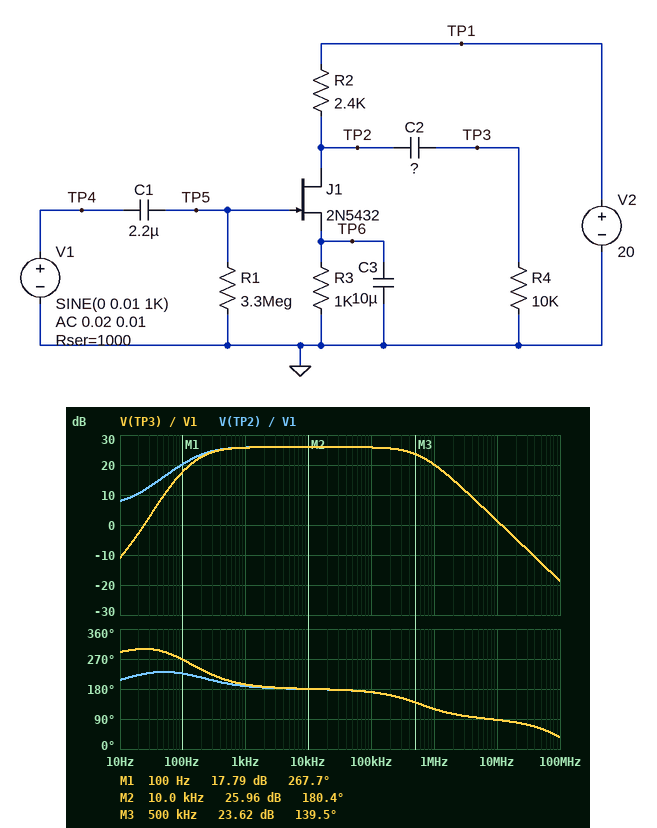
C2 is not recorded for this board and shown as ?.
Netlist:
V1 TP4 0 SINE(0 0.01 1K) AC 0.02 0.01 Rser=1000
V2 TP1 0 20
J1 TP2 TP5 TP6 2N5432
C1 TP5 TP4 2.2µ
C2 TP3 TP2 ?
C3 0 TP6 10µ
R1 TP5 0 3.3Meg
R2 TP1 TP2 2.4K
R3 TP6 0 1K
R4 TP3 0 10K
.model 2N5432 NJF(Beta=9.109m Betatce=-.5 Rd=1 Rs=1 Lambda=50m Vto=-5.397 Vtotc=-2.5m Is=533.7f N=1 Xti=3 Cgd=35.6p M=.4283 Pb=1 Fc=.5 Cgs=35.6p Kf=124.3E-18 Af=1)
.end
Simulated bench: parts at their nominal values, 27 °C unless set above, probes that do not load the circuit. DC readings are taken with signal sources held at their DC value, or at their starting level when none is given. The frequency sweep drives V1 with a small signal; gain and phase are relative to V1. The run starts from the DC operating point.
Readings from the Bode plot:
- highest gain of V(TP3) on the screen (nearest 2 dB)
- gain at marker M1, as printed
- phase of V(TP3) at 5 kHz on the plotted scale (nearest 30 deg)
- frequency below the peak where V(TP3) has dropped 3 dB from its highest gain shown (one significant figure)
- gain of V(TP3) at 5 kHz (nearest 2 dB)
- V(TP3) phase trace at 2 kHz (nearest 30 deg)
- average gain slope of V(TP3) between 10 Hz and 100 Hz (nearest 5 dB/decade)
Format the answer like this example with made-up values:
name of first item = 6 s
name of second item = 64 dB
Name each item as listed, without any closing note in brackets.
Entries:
highest gain of V(TP3) on the screen = 26 dB
gain at marker M1, as printed = 17.79 dB
phase of V(TP3) at 5 kHz on the plotted scale = 180 deg
frequency below the peak where V(TP3) has dropped 3 dB from its highest gain shown = 200 Hz
gain of V(TP3) at 5 kHz = 26 dB
V(TP3) phase trace at 2 kHz = 180 deg
average gain slope of V(TP3) between 10 Hz and 100 Hz = 30 dB/decade
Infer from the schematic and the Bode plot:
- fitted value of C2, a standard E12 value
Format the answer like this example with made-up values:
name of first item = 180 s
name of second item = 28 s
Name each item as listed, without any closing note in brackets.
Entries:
fitted value of C2, a standard E12 value = 180 nF
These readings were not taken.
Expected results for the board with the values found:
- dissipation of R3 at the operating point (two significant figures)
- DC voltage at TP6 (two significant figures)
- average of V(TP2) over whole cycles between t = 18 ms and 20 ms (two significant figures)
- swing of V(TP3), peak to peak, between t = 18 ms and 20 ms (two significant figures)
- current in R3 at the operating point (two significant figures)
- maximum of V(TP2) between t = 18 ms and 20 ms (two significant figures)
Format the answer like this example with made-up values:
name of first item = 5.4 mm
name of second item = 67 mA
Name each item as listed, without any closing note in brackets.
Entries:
dissipation of R3 at the operating point = 22 mW
DC voltage at TP6 = 4.7 V
average of V(TP2) over whole cycles between t = 18 ms and 20 ms = 8.6 V
swing of V(TP3), peak to peak, between t = 18 ms and 20 ms = 390 mV
current in R3 at the operating point = 4.7 mA
maximum of V(TP2) between t = 18 ms and 20 ms = 8.8 V
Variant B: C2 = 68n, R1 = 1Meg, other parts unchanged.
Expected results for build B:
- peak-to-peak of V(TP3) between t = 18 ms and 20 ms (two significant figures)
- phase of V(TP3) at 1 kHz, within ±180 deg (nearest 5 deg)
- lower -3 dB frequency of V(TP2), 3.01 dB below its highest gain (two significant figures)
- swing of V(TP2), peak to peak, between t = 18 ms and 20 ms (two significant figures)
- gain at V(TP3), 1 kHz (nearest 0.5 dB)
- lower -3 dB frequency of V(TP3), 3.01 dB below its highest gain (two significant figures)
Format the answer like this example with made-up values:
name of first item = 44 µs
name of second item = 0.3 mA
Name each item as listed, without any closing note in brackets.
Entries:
peak-to-peak of V(TP3) between t = 18 ms and 20 ms = 380 mV
phase of V(TP3) at 1 kHz, within ±180 deg = -160 deg
lower -3 dB frequency of V(TP2), 3.01 dB below its highest gain = 150 Hz
swing of V(TP2), peak to peak, between t = 18 ms and 20 ms = 390 mV
gain at V(TP3), 1 kHz = 25.5 dB
lower -3 dB frequency of V(TP3), 3.01 dB below its highest gain = 300 Hz
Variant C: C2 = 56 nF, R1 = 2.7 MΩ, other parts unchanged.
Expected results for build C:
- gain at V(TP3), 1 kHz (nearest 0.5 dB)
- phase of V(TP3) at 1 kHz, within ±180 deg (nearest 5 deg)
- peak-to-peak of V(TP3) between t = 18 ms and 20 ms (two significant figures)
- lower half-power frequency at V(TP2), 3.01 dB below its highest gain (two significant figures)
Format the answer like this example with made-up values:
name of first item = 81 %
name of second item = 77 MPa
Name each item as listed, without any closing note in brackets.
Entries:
gain at V(TP3), 1 kHz = 25.5 dB
phase of V(TP3) at 1 kHz, within ±180 deg = -155 deg
peak-to-peak of V(TP3) between t = 18 ms and 20 ms = 380 mV
lower half-power frequency at V(TP2), 3.01 dB below its highest gain = 140 Hz
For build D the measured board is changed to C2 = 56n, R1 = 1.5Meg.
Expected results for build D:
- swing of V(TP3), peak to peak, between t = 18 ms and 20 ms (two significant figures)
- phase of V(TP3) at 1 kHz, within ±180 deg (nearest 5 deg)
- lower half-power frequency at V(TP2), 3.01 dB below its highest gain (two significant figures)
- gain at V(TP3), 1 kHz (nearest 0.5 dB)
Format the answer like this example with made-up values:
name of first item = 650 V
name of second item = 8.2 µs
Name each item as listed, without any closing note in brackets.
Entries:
swing of V(TP3), peak to peak, between t = 18 ms and 20 ms = 380 mV
phase of V(TP3) at 1 kHz, within ±180 deg = -155 deg
lower half-power frequency at V(TP2), 3.01 dB below its highest gain = 140 Hz
gain at V(TP3), 1 kHz = 25.5 dB
